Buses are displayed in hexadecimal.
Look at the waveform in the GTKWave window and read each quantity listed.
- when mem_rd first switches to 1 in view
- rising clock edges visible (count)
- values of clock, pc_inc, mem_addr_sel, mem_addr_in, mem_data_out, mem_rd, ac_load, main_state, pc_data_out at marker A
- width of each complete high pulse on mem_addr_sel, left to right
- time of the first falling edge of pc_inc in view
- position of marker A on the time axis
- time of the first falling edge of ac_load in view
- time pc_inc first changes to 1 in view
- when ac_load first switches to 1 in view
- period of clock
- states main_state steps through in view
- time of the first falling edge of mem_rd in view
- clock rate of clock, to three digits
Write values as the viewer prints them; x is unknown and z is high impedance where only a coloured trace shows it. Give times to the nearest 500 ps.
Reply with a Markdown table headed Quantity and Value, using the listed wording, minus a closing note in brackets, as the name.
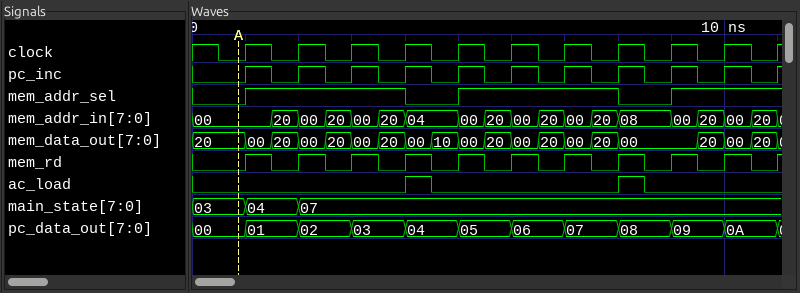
| Quantity | Value |
|---|---|
| when mem_rd first switches to 1 in view | 1000 ps |
| rising clock edges visible | 11 |
| values of clock, pc_inc, mem_addr_sel, mem_addr_in, mem_data_out, mem_rd, ac_load, main_state, pc_data_out at marker A | clock=0, pc_inc=0, mem_addr_sel=0, mem_addr_in=00, mem_data_out=20, mem_rd=0, ac_load=0, main_state=03, pc_data_out=00 |
| width of each complete high pulse on mem_addr_sel, left to right | 3000 ps, 3000 ps |
| time of the first falling edge of pc_inc in view | 1500 ps |
| position of marker A on the time axis | 1000 ps |
| time of the first falling edge of ac_load in view | 4500 ps |
| time pc_inc first changes to 1 in view | 1000 ps |
| when ac_load first switches to 1 in view | 4000 ps |
| period of clock | 1000 ps |
| states main_state steps through in view | 03, 04, 07 |
| time of the first falling edge of mem_rd in view | 1500 ps |
| clock rate of clock, to three digits | 1.00 GHz |
